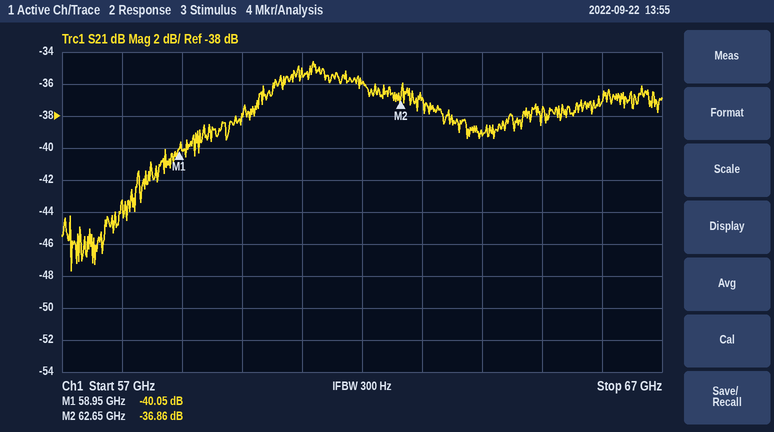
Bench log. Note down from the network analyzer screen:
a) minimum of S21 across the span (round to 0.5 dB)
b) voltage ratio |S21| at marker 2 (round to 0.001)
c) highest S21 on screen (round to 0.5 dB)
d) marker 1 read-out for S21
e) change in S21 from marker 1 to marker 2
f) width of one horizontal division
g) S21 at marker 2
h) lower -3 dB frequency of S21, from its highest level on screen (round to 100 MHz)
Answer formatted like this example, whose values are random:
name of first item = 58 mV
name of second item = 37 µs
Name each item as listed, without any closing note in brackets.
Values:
minimum of S21 across the span = -47.5 dB
voltage ratio |S21| at marker 2 = 0.014
highest S21 on screen = -34.5 dB
marker 1 read-out for S21 = -40.05 dB
change in S21 from marker 1 to marker 2 = 3.19 dB
width of one horizontal division = 1 GHz
S21 at marker 2 = -36.86 dB
lower -3 dB frequency of S21, from its highest level on screen = 60.2 GHz
